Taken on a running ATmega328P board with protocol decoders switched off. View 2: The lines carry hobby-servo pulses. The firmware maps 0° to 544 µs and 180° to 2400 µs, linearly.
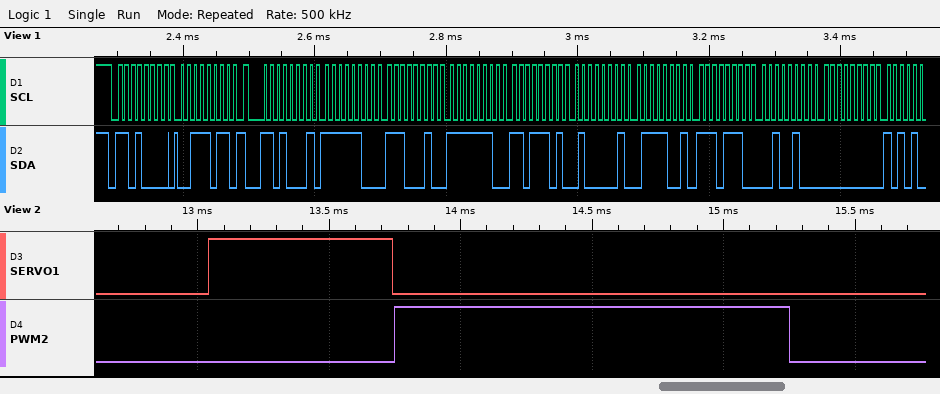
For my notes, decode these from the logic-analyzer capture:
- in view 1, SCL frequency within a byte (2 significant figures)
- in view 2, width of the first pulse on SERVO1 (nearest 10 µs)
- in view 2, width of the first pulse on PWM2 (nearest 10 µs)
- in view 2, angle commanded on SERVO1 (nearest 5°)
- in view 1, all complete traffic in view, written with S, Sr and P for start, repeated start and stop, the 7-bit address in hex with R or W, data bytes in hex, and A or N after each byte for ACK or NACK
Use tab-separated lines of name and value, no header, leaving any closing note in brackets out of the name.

in view 1, SCL frequency within a byte	100 kHz
in view 2, width of the first pulse on SERVO1	700 µs
in view 2, width of the first pulse on PWM2	1500 µs
in view 2, angle commanded on SERVO1	15°
in view 1, all complete traffic in view, written with S, Sr and P for start, repeated start and stop, the 7-bit address in hex with R or W, data bytes in hex, and A or N after each byte for ACK or NACK	S 68W A 3B A Sr 68R A FC A E2 A FE A DD A 41 A 79 A EE A 24 A 00 A
